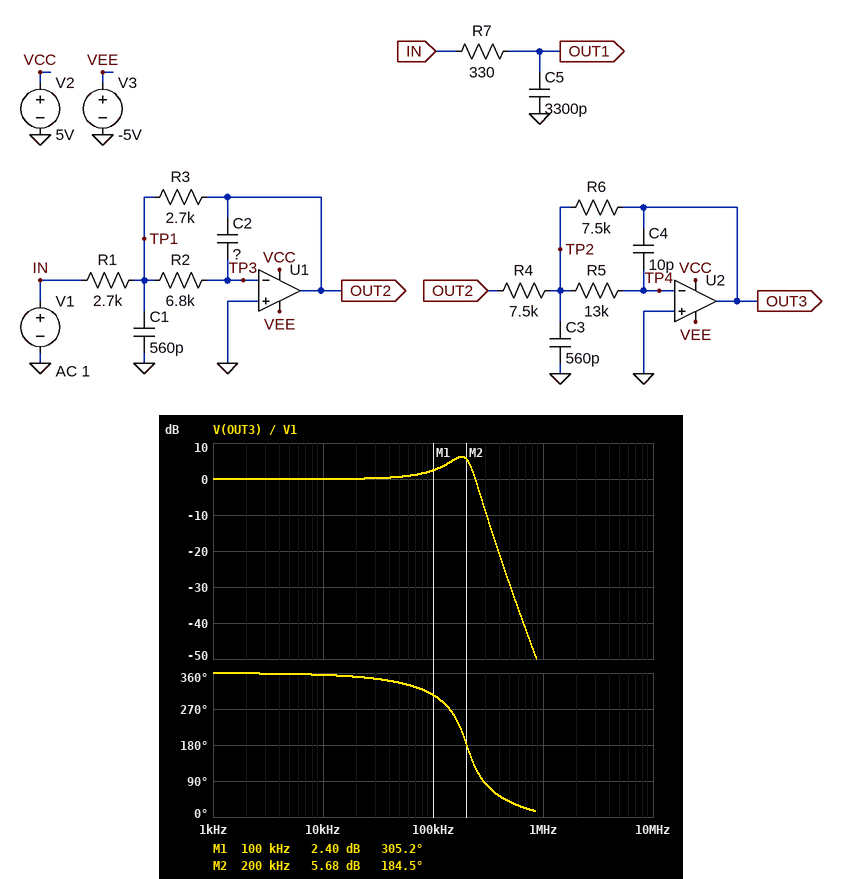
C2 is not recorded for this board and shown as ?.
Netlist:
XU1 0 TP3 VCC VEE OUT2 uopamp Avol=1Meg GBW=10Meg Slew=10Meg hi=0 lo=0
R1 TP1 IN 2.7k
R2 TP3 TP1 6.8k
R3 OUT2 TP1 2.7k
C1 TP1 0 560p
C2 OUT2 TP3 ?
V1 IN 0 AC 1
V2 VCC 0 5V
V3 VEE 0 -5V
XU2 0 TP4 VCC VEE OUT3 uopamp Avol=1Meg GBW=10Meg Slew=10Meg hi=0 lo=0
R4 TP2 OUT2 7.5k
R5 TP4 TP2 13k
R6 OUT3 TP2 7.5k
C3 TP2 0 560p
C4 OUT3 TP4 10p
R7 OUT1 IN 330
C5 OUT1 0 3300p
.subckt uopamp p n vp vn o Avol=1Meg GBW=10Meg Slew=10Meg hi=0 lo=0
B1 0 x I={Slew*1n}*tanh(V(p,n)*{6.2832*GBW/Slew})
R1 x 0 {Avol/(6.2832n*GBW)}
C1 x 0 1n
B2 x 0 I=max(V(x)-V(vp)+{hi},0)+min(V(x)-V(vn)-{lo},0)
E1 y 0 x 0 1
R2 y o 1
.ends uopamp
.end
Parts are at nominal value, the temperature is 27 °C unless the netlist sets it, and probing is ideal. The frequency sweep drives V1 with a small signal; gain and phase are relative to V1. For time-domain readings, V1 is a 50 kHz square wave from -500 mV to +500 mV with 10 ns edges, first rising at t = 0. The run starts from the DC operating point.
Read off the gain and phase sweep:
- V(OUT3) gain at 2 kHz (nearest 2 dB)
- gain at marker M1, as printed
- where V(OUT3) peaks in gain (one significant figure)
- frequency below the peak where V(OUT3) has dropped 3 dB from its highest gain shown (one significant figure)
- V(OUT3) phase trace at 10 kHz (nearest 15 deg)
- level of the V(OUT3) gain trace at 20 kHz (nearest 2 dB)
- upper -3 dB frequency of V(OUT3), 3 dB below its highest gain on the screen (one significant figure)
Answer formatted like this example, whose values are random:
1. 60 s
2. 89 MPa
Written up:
1. 0 dB
2. 2.40 dB
3. 200 kHz
4. 100 kHz
5. 360 deg
6. 0 dB
7. 200 kHz
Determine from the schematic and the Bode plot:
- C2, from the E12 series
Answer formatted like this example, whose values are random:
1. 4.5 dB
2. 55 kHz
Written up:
1. 56 pF
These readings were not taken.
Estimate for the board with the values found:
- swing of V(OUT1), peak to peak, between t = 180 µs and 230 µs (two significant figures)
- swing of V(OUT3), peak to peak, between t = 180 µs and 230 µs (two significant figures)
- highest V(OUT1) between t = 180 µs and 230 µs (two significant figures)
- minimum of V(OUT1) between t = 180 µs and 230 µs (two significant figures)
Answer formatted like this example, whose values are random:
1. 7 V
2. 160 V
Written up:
1. 1.0 V
2. 1.9 V
3. 500 mV
4. -500 mV
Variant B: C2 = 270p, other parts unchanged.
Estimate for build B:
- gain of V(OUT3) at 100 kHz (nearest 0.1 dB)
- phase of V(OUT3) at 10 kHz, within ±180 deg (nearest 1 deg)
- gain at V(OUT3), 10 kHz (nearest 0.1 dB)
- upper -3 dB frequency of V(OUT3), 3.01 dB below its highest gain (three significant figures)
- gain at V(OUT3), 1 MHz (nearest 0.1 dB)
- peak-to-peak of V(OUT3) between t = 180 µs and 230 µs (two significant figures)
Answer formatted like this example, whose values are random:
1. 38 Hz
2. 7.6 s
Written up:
1. -6.8 dB
2. -17 deg
3. -0.2 dB
4. 45.6 kHz
5. -68.5 dB
6. 870 mV
